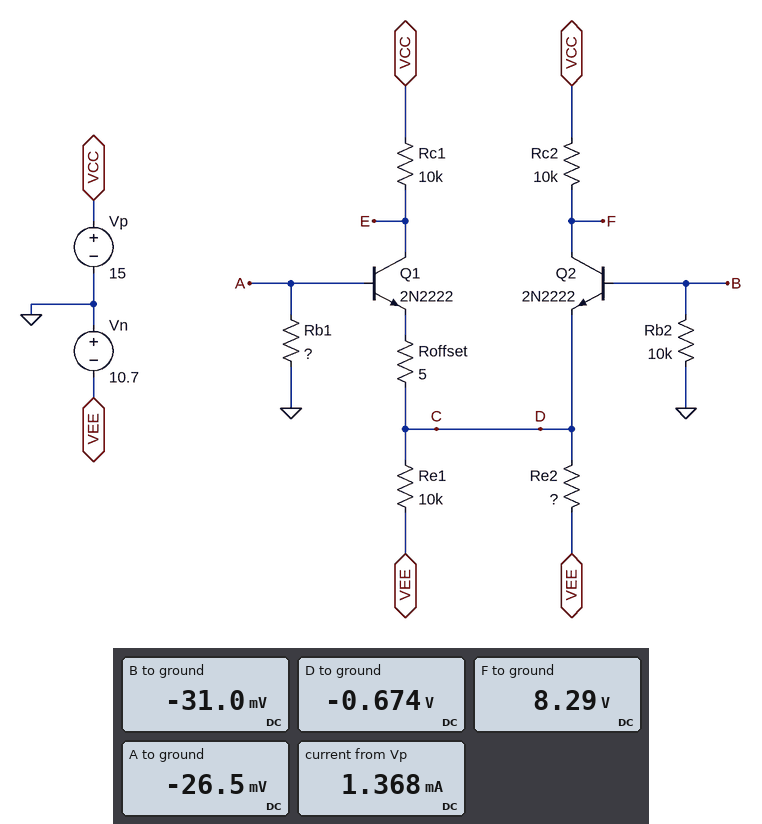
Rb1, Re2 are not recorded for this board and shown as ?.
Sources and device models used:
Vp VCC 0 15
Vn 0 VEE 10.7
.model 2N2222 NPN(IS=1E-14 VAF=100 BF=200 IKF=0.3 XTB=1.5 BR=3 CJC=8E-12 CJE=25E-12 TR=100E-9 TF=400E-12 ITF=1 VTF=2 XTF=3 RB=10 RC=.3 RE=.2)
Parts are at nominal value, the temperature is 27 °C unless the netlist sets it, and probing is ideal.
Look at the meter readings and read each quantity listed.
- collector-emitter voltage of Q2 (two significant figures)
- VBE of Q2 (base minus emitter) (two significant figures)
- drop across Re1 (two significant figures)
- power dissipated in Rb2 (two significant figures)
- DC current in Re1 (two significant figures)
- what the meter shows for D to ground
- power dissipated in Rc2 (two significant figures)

9.0 V
640 mV
10 V
96 nW
1.0 mA
-0.674 V
4.5 mW
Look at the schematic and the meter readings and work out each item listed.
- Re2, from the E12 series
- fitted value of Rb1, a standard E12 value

27 kΩ
8.2 kΩ
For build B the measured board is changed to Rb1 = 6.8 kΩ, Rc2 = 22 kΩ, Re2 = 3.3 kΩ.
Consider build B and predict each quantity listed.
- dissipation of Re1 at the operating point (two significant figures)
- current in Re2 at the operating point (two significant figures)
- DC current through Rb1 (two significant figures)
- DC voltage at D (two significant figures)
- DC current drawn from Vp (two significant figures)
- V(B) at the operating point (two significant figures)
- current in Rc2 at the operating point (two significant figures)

6.1 mW
2.4 mA
320 µA
-2.9 V
2.6 mA
-2.2 V
810 µA
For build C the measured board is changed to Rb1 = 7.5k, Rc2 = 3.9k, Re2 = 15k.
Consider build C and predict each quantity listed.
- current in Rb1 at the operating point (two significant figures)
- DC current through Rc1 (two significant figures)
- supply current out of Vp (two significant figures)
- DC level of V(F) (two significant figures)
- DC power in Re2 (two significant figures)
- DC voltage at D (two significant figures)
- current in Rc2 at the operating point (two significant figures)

4.0 µA
850 µA
1.7 mA
12 V
6.7 mW
-680 mV
810 µA
